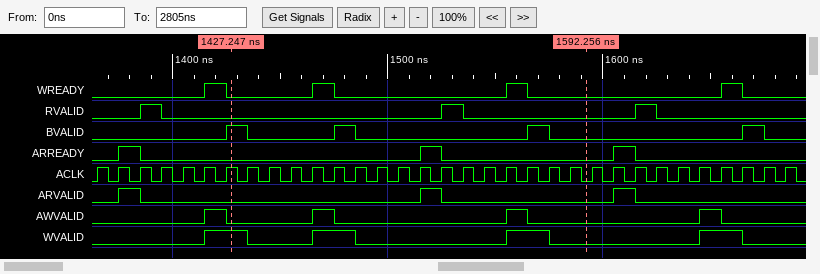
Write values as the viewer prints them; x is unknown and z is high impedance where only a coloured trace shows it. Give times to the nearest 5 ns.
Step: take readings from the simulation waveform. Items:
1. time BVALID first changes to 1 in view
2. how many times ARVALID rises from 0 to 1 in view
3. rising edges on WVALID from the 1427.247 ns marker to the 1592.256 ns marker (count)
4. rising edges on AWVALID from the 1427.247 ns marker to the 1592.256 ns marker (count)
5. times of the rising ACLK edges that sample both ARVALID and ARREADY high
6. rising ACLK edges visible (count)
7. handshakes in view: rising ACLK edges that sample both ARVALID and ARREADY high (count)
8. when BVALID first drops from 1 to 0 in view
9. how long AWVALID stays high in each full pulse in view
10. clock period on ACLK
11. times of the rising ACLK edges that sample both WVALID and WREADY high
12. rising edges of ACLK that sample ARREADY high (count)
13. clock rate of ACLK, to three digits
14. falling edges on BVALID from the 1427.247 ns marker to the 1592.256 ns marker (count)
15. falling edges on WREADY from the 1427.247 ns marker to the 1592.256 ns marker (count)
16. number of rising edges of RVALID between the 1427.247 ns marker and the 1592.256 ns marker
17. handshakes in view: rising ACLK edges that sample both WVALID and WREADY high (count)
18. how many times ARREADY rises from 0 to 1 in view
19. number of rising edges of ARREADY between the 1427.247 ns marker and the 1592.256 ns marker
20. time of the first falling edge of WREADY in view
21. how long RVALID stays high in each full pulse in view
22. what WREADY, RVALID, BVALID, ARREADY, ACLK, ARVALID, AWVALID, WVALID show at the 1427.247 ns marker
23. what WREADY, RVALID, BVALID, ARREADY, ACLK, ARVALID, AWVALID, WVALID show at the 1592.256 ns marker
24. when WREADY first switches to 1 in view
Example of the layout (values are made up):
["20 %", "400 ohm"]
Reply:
["1425 ns", "3", "2", "2", "1385 ns, 1525 ns, 1615 ns", "33", "3", "1435 ns", "10 ns, 10 ns, 10 ns, 10 ns", "10 ns", "1425 ns, 1475 ns, 1565 ns, 1665 ns", "3", "100 MHz", "3", "2", "1", "4", "3", "1", "1425 ns", "10 ns, 10 ns, 10 ns", "WREADY=0, RVALID=0, BVALID=1, ARREADY=0, ACLK=1, ARVALID=0, AWVALID=0, WVALID=1", "WREADY=0, RVALID=0, BVALID=0, ARREADY=0, ACLK=0, ARVALID=0, AWVALID=0, WVALID=0", "1415 ns"]
